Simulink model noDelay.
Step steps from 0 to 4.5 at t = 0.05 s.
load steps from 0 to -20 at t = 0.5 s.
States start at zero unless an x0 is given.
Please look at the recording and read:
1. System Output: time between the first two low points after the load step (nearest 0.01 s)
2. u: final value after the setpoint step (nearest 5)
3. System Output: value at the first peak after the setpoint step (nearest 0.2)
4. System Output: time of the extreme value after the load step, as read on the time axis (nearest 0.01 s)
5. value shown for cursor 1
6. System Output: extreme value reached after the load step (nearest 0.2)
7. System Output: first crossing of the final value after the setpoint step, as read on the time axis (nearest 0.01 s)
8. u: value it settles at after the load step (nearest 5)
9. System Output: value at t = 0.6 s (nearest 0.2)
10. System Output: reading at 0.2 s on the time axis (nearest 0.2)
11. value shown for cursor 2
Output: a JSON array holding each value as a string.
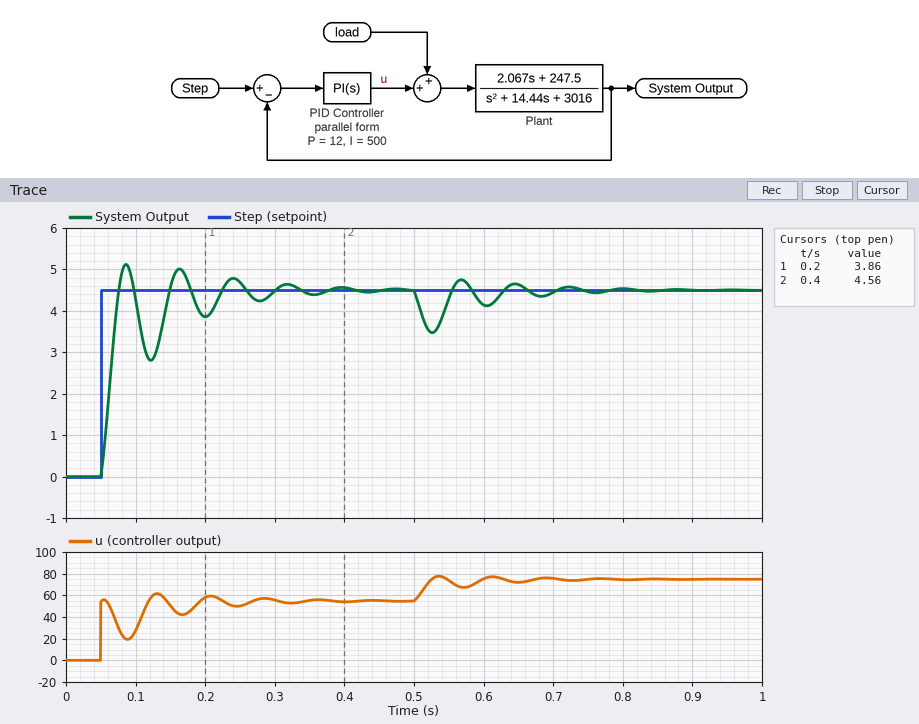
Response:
["0.08 s", "55", "5.2", "0.53 s", "3.86", "3.4", "0.08 s", "75", "4.2", "3.8", "4.56"]
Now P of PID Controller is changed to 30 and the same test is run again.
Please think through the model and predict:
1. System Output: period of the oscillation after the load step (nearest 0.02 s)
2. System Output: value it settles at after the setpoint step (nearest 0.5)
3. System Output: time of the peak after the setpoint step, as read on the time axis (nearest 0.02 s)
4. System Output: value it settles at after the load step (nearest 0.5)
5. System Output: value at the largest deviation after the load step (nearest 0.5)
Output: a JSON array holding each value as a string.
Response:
["0.06 s", "4.5", "0.08 s", "4.5", "4.0"]
